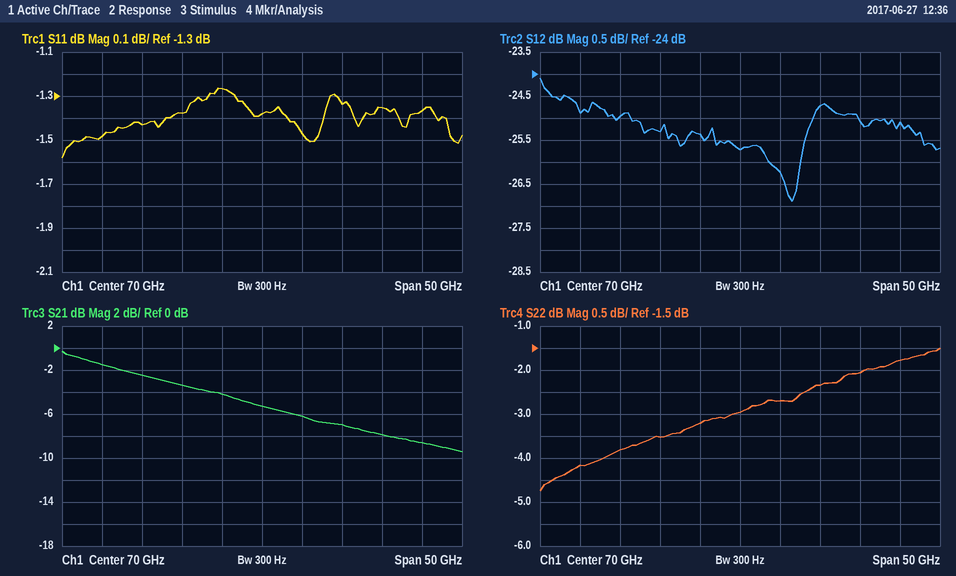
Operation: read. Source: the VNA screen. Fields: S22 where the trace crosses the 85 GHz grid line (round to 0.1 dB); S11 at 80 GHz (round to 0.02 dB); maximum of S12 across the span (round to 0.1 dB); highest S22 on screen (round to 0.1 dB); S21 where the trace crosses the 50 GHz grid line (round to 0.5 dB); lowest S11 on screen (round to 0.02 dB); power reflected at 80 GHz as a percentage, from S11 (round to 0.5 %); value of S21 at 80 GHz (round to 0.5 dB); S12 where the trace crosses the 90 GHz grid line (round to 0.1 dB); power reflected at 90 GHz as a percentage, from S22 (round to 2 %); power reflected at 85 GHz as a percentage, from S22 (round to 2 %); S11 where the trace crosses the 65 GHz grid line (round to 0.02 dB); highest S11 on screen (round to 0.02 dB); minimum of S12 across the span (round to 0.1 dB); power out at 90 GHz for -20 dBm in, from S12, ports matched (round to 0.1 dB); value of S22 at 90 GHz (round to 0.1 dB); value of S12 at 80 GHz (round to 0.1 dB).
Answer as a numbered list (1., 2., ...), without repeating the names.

1. -2.1 dB
2. -1.34 dB
3. -24.1 dB
4. -1.5 dB
5. -1.5 dB
6. -1.58 dB
7. 73.5 %
8. -7.0 dB
9. -25.1 dB
10. 66 %
11. 62 %
12. -1.26 dB
13. -1.26 dB
14. -26.9 dB
15. -45.1 dBm
16. -1.8 dB
17. -24.7 dB
